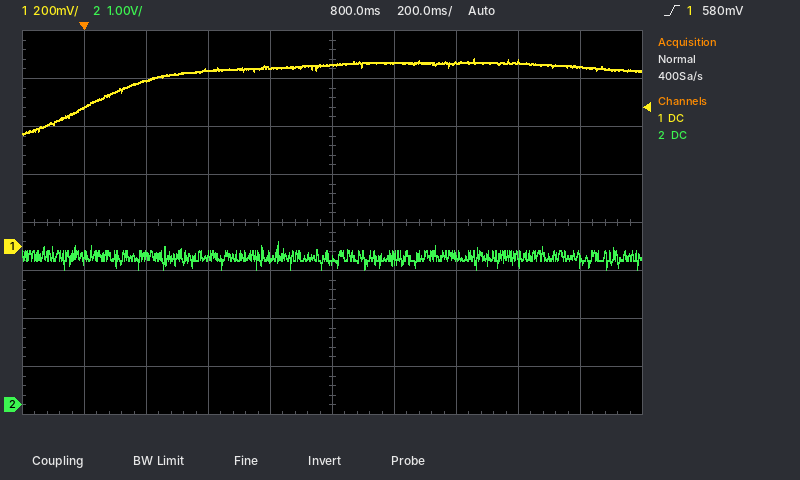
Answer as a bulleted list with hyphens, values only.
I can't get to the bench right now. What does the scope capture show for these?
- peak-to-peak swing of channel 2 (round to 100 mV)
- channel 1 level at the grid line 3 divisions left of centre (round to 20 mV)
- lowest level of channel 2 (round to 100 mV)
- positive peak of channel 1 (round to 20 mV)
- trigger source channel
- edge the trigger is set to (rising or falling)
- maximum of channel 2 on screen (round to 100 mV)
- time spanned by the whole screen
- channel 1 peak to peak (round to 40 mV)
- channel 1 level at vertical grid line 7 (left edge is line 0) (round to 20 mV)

- 600 mV
- 700 mV
- 2.8 V
- 780 mV
- channel 1
- rising
- 3.4 V
- 2 s
- 320 mV
- 760 mV
